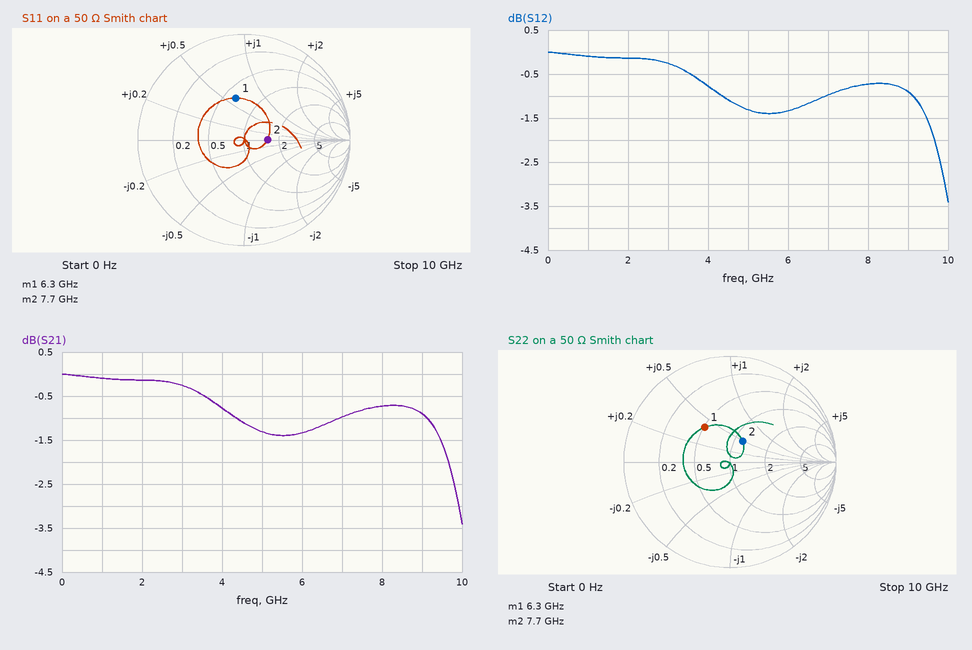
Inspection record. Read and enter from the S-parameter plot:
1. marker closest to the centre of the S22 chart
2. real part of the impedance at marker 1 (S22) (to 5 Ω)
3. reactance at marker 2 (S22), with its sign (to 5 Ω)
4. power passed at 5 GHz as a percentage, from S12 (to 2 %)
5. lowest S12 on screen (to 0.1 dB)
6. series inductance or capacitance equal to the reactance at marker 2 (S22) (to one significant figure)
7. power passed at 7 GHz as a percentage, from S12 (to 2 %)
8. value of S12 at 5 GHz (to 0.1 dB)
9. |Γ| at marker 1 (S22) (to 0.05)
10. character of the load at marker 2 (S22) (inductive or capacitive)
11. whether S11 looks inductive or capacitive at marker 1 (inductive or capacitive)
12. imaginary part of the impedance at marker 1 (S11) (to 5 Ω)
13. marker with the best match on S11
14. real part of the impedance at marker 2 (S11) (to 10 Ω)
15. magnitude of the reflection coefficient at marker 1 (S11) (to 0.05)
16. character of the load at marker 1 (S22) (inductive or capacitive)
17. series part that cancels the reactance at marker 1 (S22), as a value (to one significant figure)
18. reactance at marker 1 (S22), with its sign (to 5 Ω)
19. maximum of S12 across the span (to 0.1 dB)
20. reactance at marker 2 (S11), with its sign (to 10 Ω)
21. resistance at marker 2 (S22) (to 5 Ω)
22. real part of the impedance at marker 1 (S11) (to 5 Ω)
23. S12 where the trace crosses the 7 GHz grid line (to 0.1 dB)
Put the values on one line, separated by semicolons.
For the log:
marker 2; 25 Ω; +25 Ω; 74 %; -3.4 dB; 500 pH; 80 %; -1.3 dB; 0.40; inductive; inductive; +30 Ω; marker 2; 80 Ω; 0.40; inductive; 1 pF; +20 Ω; 0.0 dB; 0 Ω; 60 Ω; 30 Ω; -1.0 dB
